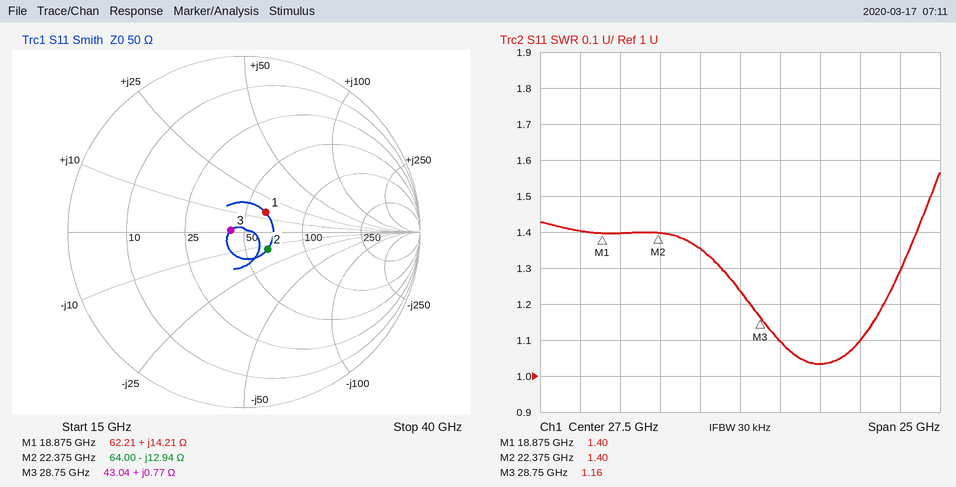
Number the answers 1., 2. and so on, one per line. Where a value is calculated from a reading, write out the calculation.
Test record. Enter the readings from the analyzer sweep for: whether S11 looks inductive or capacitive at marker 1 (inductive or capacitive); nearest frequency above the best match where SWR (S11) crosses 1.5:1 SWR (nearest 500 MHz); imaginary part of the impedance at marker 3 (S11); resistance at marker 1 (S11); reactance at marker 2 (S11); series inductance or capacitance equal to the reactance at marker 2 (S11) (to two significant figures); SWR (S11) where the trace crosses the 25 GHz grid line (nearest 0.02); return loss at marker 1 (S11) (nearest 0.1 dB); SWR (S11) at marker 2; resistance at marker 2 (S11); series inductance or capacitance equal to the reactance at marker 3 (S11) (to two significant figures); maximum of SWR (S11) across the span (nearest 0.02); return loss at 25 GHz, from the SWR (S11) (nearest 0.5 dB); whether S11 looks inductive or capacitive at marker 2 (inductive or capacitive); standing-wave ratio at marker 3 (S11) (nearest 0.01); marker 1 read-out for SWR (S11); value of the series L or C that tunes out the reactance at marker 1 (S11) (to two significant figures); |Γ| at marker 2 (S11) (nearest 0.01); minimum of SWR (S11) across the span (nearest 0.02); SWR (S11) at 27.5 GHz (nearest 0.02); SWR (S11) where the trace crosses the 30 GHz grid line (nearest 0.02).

1. inductive
2. 39.5 GHz
3. +0.77 Ω
4. 62.21 Ω
5. -12.94 Ω
6. C = 1/(2π × 22.375 GHz × 12.94 Ω) ≈ 550 fF
7. 1.36
8. 15.6 dB
9. 1.40
10. 64.00 Ω
11. L = 0.77 Ω/(2π × 28.75 GHz) ≈ 4.3 pH
12. 1.56
13. −20 log10((1.36 − 1)/(1.36 + 1)) ≈ 16.3 dB, so 16.5 dB to the nearest 0.5 dB
14. capacitive
15. 1.16
16. 1.40
17. C = 1/(2π × 18.875 GHz × 14.21 Ω) ≈ 593 fF, so 590 fF to two significant figures
18. 0.17
19. 1.04
20. 1.24
21. 1.10
